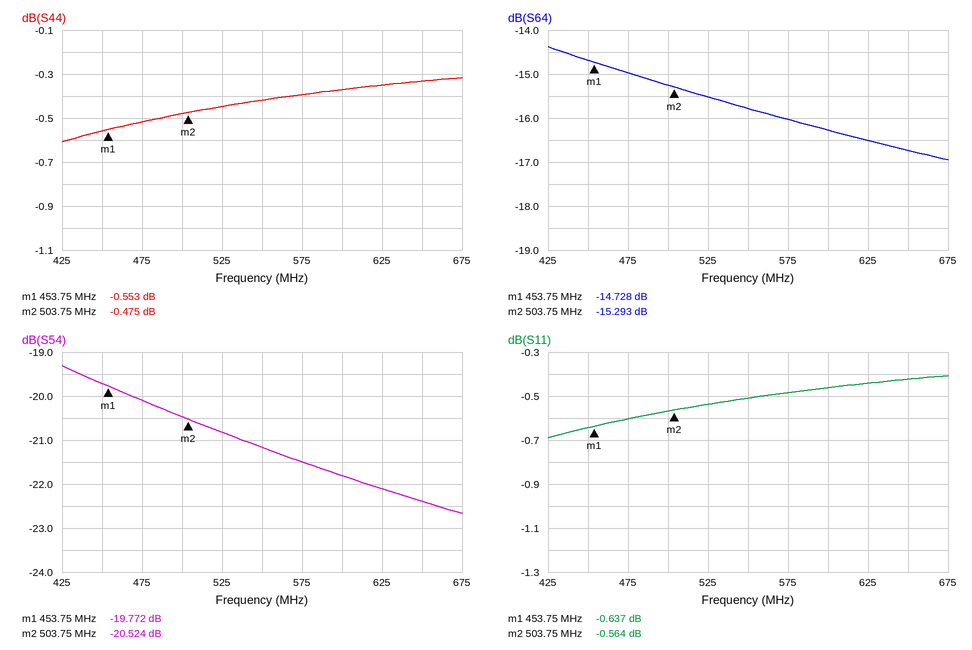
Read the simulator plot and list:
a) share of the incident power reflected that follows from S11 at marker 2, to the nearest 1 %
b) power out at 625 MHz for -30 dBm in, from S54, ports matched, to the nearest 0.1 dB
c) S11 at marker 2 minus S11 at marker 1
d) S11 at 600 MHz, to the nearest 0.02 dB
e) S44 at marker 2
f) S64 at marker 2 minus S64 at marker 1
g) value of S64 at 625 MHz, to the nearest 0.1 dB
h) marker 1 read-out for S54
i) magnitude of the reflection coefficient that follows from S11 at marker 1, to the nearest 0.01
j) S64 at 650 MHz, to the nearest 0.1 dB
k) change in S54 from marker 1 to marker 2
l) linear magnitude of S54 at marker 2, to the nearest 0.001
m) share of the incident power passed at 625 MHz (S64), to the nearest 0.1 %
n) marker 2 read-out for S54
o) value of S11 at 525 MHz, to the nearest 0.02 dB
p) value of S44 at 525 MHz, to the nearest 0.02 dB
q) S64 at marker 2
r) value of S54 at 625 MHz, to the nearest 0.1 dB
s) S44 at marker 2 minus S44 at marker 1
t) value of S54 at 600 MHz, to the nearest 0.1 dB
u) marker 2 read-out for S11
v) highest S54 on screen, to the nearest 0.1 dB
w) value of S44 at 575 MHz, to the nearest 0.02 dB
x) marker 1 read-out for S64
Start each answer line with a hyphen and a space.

- 88 %
- -52.1 dBm
- 0.073 dB
- -0.46 dB
- -0.475 dB
- -0.565 dB
- -16.5 dB
- -19.772 dB
- 0.93
- -16.7 dB
- -0.752 dB
- 0.094
- 2.2 %
- -20.524 dB
- -0.54 dB
- -0.44 dB
- -15.293 dB
- -22.1 dB
- 0.078 dB
- -21.8 dB
- -0.564 dB
- -19.3 dB
- -0.40 dB
- -14.728 dB
